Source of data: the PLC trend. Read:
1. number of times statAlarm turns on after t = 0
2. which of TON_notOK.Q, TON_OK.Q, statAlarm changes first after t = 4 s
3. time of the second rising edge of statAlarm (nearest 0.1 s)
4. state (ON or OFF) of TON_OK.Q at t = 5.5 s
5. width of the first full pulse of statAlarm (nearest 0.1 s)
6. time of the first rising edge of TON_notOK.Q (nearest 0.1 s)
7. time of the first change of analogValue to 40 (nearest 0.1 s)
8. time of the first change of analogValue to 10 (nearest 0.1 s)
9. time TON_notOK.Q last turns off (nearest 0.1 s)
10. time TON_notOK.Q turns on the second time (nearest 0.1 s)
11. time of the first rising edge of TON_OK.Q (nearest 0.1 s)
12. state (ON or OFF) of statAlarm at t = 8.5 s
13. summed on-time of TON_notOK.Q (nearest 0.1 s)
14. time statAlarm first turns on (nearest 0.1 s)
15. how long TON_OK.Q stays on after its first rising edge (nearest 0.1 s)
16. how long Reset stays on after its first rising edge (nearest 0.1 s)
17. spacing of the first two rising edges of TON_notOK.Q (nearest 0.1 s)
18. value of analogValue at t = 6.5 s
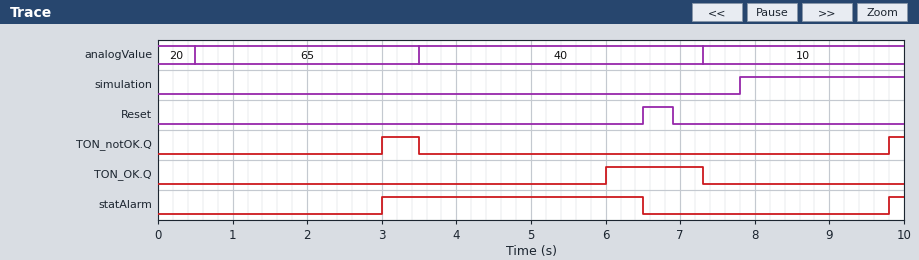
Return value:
2
TON_OK.Q
9.8 s
OFF
3.5 s
3.0 s
3.5 s
7.3 s
3.5 s
9.8 s
6.0 s
OFF
0.7 s
3.0 s
1.3 s
0.4 s
6.8 s
40
